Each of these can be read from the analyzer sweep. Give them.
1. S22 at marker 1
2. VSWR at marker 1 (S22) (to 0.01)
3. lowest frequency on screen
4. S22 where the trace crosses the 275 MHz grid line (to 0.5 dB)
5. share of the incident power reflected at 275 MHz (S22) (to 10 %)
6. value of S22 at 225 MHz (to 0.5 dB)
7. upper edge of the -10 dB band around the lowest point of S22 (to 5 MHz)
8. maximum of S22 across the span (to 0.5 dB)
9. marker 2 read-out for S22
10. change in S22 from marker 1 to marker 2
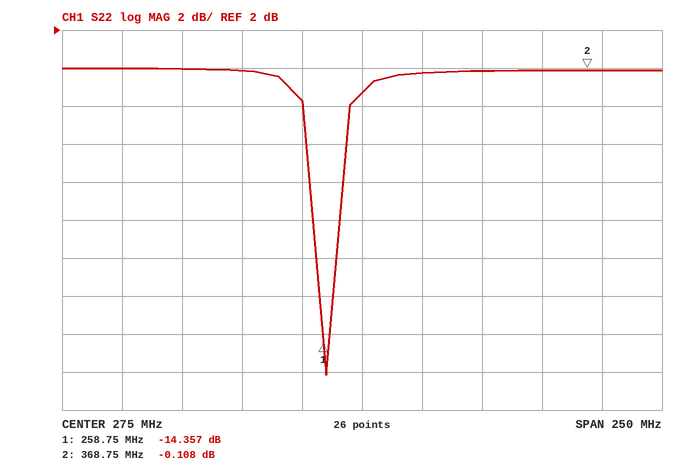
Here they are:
-14.357 dB
1.47
150 MHz
-1.5 dB
70 %
0.0 dB
265 MHz
0.0 dB
-0.108 dB
14.249 dB
